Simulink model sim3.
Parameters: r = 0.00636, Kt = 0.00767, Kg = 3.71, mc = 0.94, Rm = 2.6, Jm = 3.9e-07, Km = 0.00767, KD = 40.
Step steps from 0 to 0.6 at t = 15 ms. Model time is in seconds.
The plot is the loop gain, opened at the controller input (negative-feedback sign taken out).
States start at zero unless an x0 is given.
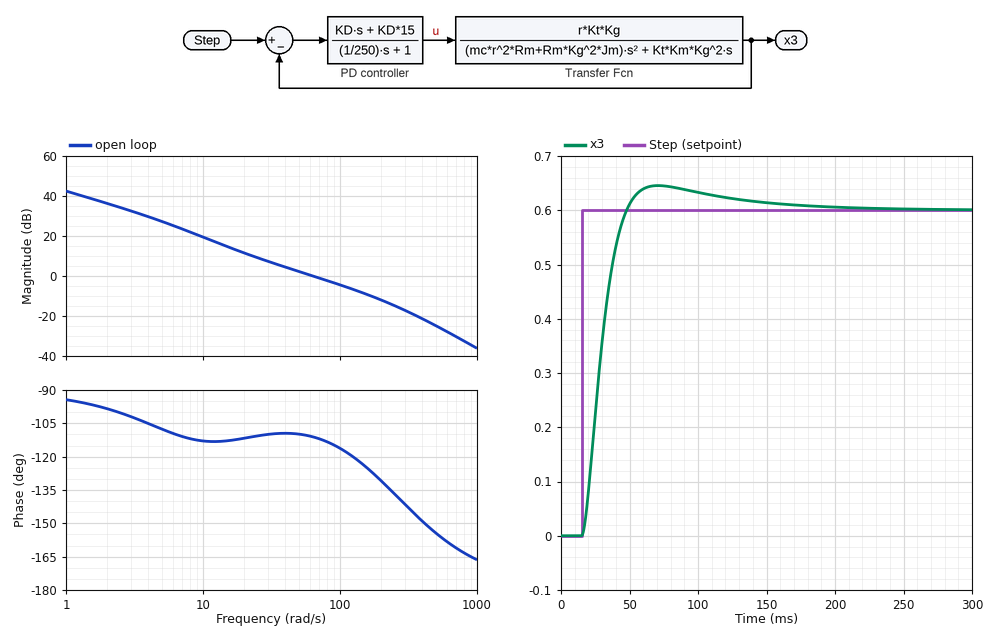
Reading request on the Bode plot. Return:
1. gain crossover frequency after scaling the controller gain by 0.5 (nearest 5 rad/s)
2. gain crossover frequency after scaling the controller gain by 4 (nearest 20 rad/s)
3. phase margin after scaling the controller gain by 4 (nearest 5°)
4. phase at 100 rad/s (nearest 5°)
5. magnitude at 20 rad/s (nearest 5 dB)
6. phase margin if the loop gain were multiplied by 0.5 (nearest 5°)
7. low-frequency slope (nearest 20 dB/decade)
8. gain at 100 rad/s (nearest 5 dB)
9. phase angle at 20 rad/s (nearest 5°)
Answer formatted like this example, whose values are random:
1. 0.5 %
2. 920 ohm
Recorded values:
1. 35 rad/s
2. 200 rad/s
3. 50°
4. -115°
5. 10 dB
6. 70°
7. -20 dB/decade
8. -5 dB
9. -110°
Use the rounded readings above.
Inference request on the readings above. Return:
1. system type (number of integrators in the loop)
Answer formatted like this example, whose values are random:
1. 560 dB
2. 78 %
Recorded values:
1. 1
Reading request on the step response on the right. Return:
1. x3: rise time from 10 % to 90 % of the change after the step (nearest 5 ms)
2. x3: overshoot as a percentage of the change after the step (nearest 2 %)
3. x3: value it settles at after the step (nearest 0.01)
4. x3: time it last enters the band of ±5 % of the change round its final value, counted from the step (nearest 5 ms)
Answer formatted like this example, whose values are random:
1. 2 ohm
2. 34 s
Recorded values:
1. 20 ms
2. 8 %
3. 0.60
4. 90 ms
